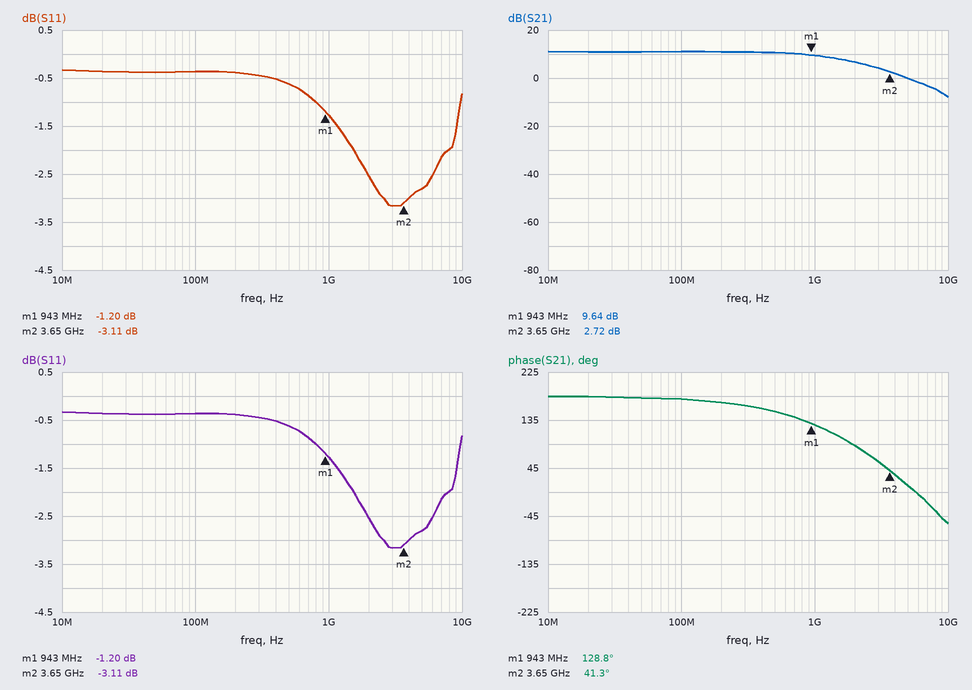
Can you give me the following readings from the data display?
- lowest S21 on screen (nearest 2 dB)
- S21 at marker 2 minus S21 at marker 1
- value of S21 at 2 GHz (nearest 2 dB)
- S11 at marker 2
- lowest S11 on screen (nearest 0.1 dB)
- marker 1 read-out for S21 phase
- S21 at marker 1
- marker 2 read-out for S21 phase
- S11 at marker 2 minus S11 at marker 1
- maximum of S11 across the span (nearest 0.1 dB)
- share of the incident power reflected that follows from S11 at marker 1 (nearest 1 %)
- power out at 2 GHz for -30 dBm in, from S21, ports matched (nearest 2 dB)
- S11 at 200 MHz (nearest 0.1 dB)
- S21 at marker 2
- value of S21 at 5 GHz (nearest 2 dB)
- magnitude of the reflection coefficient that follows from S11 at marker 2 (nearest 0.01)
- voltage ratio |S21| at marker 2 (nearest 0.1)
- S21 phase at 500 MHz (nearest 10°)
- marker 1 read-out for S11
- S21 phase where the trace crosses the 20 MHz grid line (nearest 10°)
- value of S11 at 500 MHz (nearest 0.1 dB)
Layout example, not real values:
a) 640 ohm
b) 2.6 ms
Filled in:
a) -8 dB
b) -6.92 dB
c) 6 dB
d) -3.11 dB
e) -3.2 dB
f) 128.8°
g) 9.64 dB
h) 41.3°
i) -1.91 dB
j) -0.3 dB
k) 76 %
l) -24 dBm
m) -0.4 dB
n) 2.72 dB
o) 0 dB
p) 0.70
q) 1.4
r) 150°
s) -1.20 dB
t) 180°
u) -0.6 dB
